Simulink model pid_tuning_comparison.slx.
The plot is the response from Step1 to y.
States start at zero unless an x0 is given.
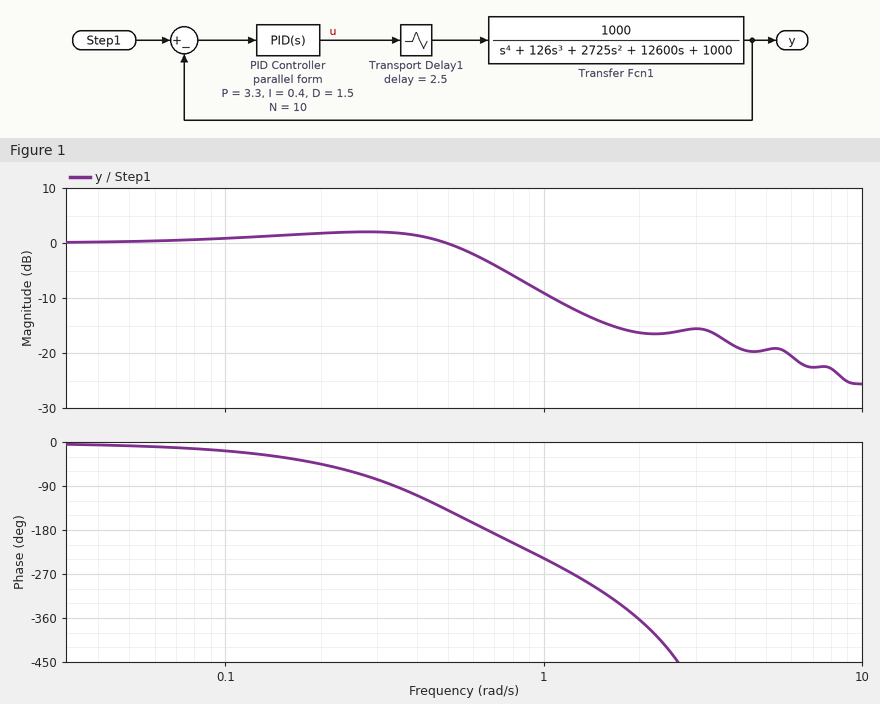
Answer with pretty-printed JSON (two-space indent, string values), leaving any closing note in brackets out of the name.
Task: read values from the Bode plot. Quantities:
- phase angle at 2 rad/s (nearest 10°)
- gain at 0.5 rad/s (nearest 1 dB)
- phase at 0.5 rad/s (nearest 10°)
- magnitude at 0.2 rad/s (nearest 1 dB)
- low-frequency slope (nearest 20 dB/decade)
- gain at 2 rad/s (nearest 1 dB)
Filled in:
{
  "phase angle at 2 rad/s": "-360°",
  "gain at 0.5 rad/s": "0 dB",
  "phase at 0.5 rad/s": "-140°",
  "magnitude at 0.2 rad/s": "2 dB",
  "low-frequency slope": "0 dB/decade",
  "gain at 2 rad/s": "-16 dB"
}
